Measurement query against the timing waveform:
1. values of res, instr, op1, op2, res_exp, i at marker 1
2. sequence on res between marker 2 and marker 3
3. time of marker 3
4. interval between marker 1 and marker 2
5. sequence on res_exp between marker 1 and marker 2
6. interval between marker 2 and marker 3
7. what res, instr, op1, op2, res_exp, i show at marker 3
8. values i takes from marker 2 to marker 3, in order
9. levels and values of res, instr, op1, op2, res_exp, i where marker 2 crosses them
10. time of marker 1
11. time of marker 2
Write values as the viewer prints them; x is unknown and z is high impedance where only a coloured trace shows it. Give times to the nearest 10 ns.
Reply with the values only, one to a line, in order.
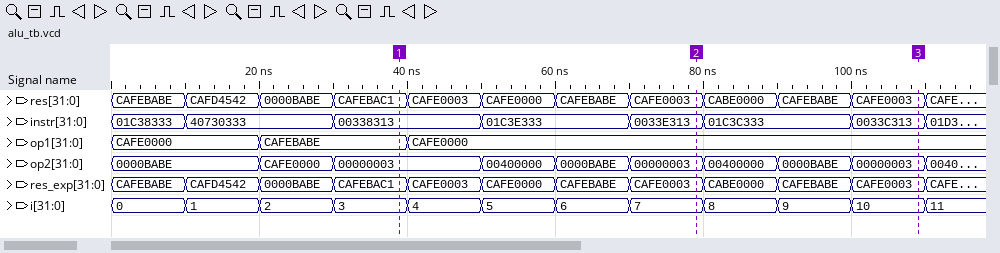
res=CAFEBAC1, instr=00338313, op1=CAFEBABE, op2=00000003, res_exp=CAFEBAC1, i=3
CAFE0003, CABE0000, CAFEBABE, CAFE0003
110 ns
40 ns
CAFEBAC1, CAFE0003, CAFE0000, CAFEBABE, CAFE0003
30 ns
res=CAFE0003, instr=0033C313, op1=CAFE0000, op2=00000003, res_exp=CAFE0003, i=10
7, 8, 9, 10
res=CAFE0003, instr=0033E313, op1=CAFE0000, op2=00000003, res_exp=CAFE0003, i=7
40 ns
80 ns
